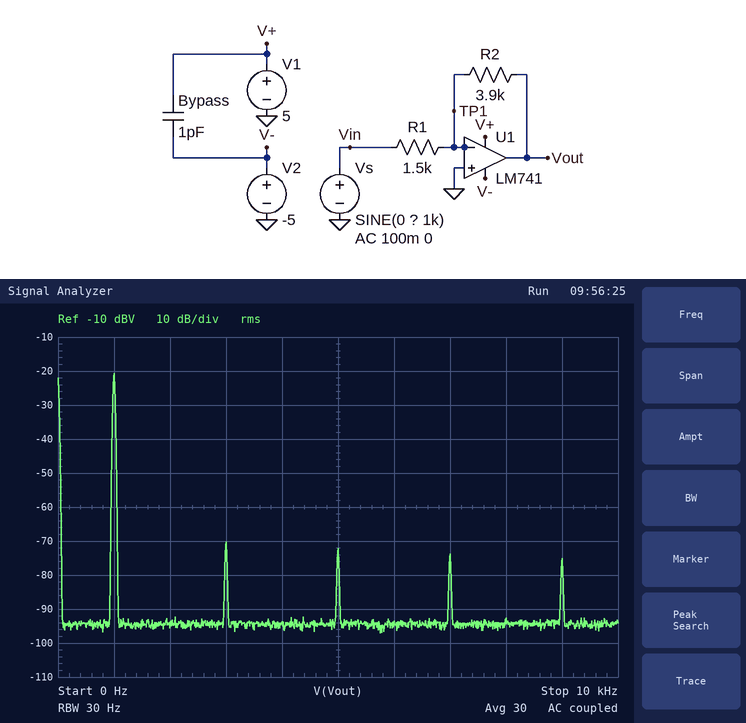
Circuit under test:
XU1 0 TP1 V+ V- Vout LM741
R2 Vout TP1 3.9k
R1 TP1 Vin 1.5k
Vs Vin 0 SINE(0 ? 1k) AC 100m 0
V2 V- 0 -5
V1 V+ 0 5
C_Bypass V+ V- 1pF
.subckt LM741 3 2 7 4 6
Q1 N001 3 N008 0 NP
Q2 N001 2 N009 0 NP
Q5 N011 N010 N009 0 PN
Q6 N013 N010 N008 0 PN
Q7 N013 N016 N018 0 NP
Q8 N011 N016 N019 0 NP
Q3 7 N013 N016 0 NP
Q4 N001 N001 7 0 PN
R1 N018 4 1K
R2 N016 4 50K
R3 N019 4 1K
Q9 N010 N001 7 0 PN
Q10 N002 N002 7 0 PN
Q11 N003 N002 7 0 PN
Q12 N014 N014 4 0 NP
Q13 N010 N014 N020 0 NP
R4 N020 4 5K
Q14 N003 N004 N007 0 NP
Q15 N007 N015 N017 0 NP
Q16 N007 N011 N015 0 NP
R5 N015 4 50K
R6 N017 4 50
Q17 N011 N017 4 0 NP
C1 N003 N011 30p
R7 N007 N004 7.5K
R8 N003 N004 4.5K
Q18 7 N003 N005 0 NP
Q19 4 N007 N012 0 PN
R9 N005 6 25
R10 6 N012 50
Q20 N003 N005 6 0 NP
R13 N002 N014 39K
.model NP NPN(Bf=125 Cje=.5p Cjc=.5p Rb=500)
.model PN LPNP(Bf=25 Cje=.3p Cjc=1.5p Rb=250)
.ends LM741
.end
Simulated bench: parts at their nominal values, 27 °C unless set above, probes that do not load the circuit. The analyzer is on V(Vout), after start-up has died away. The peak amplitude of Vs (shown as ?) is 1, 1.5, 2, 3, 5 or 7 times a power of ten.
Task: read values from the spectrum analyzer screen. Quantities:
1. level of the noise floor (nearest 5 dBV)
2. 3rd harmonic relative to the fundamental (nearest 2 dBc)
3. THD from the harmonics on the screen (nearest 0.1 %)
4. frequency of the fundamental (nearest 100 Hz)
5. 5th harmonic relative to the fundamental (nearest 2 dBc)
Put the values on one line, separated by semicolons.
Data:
-95 dBV; -50 dBc; 0.5 %; 1.0 kHz; -52 dBc
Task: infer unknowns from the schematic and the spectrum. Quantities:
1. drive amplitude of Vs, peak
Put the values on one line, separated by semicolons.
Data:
50 mV
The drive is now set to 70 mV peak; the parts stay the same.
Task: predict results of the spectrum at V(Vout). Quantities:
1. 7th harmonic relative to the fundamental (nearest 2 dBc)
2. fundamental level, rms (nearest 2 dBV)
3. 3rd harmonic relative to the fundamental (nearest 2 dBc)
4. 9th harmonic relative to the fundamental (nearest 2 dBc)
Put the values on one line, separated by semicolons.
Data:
-54 dBc; -18 dBV; -52 dBc; -56 dBc
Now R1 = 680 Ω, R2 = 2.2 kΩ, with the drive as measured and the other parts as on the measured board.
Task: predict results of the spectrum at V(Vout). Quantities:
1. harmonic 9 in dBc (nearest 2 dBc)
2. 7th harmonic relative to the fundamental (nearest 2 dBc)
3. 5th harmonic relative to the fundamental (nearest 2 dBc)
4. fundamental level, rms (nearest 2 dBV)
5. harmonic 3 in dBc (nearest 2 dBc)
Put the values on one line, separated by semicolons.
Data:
-52 dBc; -50 dBc; -50 dBc; -18 dBV; -48 dBc
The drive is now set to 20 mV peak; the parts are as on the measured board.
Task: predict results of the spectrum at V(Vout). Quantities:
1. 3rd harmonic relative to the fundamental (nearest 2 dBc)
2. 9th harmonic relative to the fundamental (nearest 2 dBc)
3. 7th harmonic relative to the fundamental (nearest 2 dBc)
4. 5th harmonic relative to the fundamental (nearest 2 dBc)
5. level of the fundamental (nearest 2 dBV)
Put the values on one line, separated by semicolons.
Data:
-46 dBc; -52 dBc; -50 dBc; -48 dBc; -28 dBV
